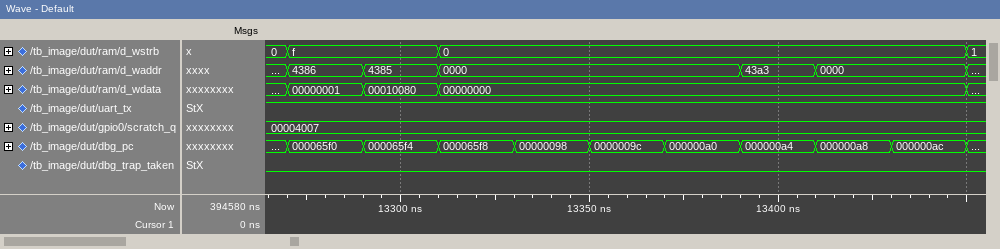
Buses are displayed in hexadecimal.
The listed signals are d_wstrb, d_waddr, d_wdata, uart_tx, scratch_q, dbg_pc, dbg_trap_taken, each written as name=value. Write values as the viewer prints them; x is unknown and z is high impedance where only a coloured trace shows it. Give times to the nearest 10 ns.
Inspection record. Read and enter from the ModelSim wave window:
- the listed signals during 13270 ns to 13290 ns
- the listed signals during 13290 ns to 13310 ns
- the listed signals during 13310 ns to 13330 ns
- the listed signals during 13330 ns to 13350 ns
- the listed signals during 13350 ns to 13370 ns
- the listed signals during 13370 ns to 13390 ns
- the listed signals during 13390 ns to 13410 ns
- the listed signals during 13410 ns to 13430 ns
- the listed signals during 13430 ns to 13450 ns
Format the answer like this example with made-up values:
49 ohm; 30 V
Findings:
d_wstrb=f, d_waddr=4386, d_wdata=00000001, uart_tx=1, scratch_q=00004007, dbg_pc=000065f0, dbg_trap_taken=0; d_wstrb=f, d_waddr=4385, d_wdata=00010080, uart_tx=1, scratch_q=00004007, dbg_pc=000065f4, dbg_trap_taken=0; d_wstrb=0, d_waddr=0000, d_wdata=00000000, uart_tx=1, scratch_q=00004007, dbg_pc=000065f8, dbg_trap_taken=0; d_wstrb=0, d_waddr=0000, d_wdata=00000000, uart_tx=1, scratch_q=00004007, dbg_pc=00000098, dbg_trap_taken=0; d_wstrb=0, d_waddr=0000, d_wdata=00000000, uart_tx=1, scratch_q=00004007, dbg_pc=0000009c, dbg_trap_taken=0; d_wstrb=0, d_waddr=0000, d_wdata=00000000, uart_tx=1, scratch_q=00004007, dbg_pc=000000a0, dbg_trap_taken=0; d_wstrb=0, d_waddr=43a3, d_wdata=00000000, uart_tx=1, scratch_q=00004007, dbg_pc=000000a4, dbg_trap_taken=0; d_wstrb=0, d_waddr=0000, d_wdata=00000000, uart_tx=1, scratch_q=00004007, dbg_pc=000000a8, dbg_trap_taken=0; d_wstrb=0, d_waddr=0000, d_wdata=00000000, uart_tx=1, scratch_q=00004007, dbg_pc=000000ac, dbg_trap_taken=0
